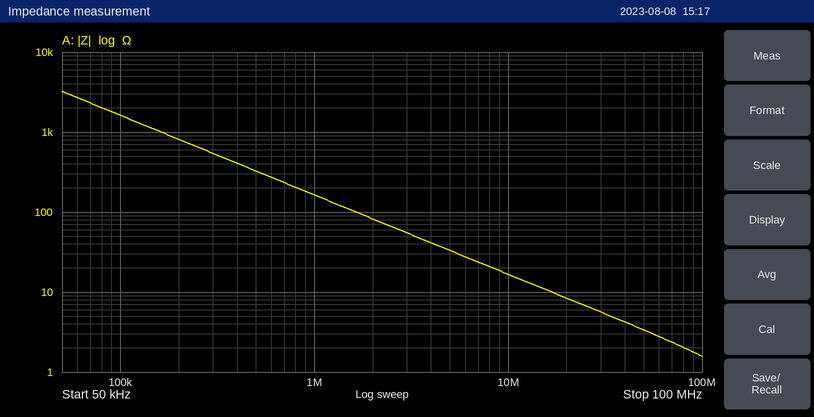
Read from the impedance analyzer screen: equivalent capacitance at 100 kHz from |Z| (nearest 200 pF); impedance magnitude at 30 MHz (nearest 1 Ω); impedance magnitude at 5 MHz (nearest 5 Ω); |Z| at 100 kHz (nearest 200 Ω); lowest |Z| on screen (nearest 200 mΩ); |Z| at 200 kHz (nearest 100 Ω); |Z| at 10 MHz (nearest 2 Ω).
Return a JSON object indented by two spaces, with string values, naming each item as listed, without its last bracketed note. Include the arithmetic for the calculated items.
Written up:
{
  "equivalent capacitance at 100 kHz from |Z|": "C = 1/(2π × 100 kHz × 1.6 kΩ) ≈ 1.0 nF",
  "impedance magnitude at 30 MHz": "6 Ω",
  "impedance magnitude at 5 MHz": "35 Ω",
  "|Z| at 100 kHz": "1.6 kΩ",
  "lowest |Z| on screen": "1.6 Ω",
  "|Z| at 200 kHz": "800 Ω",
  "|Z| at 10 MHz": "16 Ω"
}
